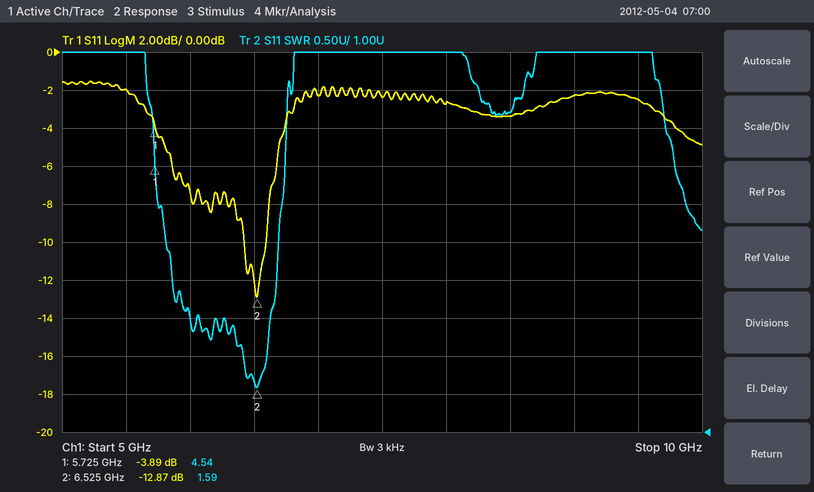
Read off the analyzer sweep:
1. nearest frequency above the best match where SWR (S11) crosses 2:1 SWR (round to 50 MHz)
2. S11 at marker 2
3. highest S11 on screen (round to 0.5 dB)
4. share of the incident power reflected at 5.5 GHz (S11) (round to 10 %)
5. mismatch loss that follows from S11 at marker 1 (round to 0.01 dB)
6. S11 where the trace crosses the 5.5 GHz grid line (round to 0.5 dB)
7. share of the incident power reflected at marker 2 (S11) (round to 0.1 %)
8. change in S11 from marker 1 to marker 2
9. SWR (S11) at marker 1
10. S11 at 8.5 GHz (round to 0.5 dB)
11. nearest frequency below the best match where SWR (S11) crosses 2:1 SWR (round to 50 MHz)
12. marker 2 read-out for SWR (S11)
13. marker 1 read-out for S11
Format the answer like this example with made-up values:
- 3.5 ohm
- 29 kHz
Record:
- 6.60 GHz
- -12.87 dB
- -1.5 dB
- 60 %
- 2.28 dB
- -2.0 dB
- 5.2 %
- -8.98 dB
- 4.54
- -3.5 dB
- 6.40 GHz
- 1.59
- -3.89 dB
